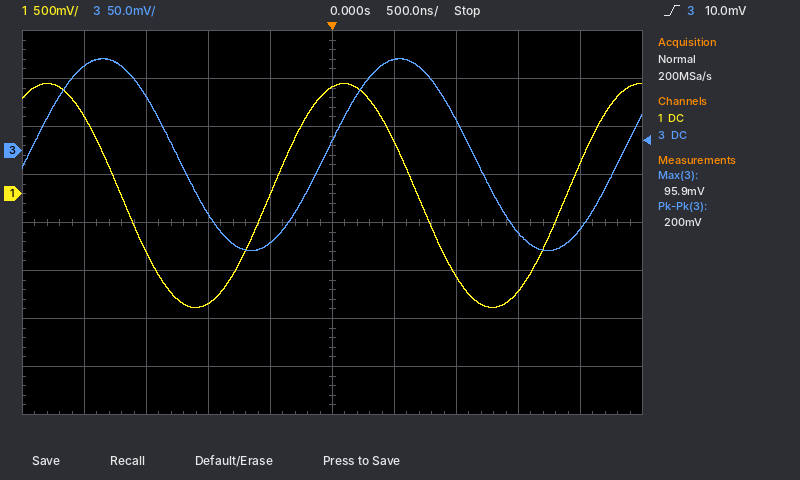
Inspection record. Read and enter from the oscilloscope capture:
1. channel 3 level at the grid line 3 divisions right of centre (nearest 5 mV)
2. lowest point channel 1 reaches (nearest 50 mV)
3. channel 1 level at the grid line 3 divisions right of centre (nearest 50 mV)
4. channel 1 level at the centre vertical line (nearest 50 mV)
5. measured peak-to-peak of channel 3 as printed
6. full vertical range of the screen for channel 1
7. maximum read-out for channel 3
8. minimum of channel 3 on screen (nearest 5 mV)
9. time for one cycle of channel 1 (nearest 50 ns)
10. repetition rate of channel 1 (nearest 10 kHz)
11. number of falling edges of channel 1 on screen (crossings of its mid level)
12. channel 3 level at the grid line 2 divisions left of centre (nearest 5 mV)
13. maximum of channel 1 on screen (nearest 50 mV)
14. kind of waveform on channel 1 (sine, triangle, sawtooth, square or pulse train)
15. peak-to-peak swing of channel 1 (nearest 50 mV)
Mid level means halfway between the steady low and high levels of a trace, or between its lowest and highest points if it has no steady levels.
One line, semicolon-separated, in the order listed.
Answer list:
-85 mV; -1.20 V; -1.00 V; 1.10 V; 200 mV; 4 V; 95.9 mV; -105 mV; 2.40 µs; 420 kHz; 2; -65 mV; 1.15 V; sine; 2.35 V
